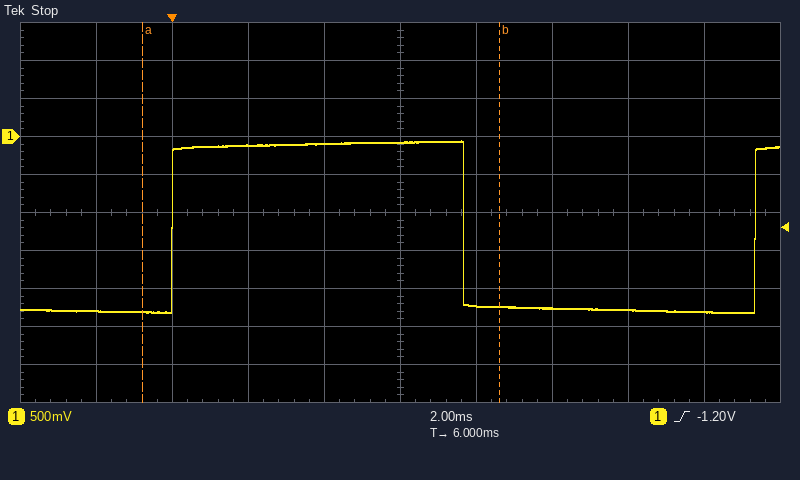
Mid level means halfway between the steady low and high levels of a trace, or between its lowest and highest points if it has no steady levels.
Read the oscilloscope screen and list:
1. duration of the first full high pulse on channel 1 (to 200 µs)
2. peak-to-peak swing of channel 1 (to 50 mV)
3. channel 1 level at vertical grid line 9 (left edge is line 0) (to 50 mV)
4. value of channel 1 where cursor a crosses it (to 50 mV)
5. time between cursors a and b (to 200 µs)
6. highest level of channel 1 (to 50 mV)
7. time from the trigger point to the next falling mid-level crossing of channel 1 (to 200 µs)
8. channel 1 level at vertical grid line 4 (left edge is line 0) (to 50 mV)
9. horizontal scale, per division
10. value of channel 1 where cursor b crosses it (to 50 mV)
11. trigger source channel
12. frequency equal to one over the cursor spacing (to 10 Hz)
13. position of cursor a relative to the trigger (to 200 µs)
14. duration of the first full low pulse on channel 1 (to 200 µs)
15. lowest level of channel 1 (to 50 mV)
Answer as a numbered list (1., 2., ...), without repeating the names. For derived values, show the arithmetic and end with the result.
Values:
1. 7.6 ms
2. -50 mV − (-2.30 V) = 2.25 V
3. -2.30 V
4. -2.30 V
5. 9.4 ms
6. -50 mV
7. 7.6 ms
8. -100 mV
9. 2 ms
10. -2.25 V
11. channel 1
12. 1 / 9.4 ms ≈ 110 Hz
13. -800 µs
14. 7.6 ms
15. -2.30 V
